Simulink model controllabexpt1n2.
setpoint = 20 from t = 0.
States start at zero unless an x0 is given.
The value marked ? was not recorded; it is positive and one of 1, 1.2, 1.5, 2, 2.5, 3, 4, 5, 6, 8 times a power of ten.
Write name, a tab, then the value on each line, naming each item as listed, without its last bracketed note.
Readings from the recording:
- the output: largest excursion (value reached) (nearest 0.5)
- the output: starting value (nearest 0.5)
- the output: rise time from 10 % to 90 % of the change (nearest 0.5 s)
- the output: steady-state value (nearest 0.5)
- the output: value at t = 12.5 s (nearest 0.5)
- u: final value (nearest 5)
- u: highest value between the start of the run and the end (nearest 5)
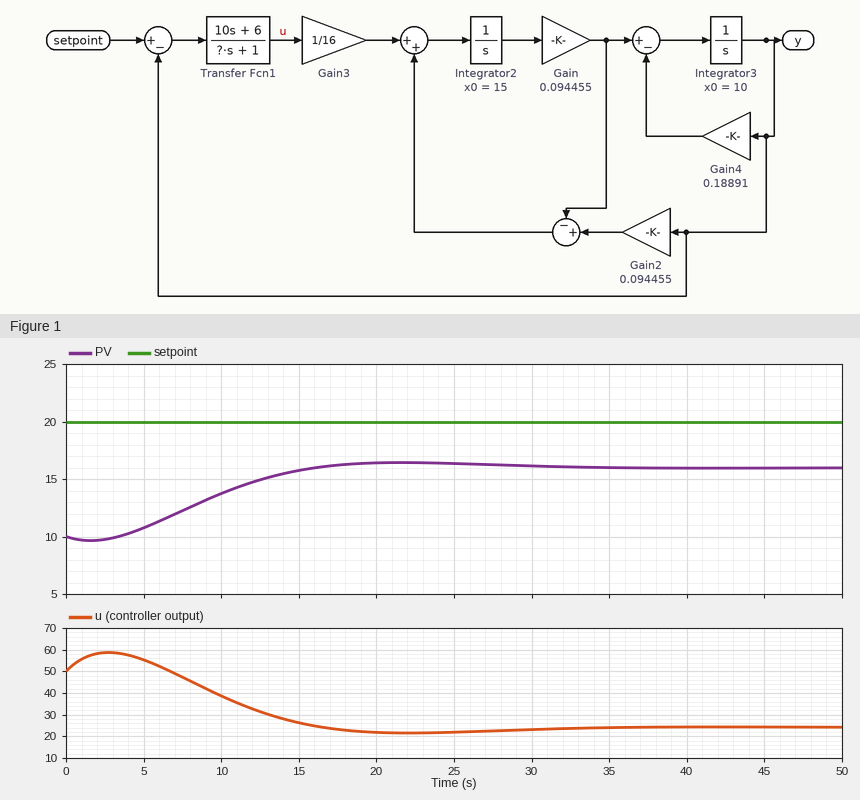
the output: largest excursion (value reached)	16.5
the output: starting value	10.0
the output: rise time from 10 % to 90 % of the change	9.0 s
the output: steady-state value	16.0
the output: value at t = 12.5 s	15.0
u: final value	25
u: highest value between the start of the run and the end	60
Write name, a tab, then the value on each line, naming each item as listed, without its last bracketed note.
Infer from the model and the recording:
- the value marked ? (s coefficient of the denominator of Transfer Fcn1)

the value marked ?	2
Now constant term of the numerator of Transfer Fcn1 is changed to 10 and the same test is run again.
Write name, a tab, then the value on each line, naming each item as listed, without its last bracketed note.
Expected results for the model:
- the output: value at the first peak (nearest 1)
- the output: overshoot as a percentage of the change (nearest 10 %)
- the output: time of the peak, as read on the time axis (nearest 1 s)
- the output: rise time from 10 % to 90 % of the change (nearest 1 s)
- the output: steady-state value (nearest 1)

the output: value at the first peak	19
the output: overshoot as a percentage of the change	20 %
the output: time of the peak, as read on the time axis	16 s
the output: rise time from 10 % to 90 % of the change	6 s
the output: steady-state value	17
